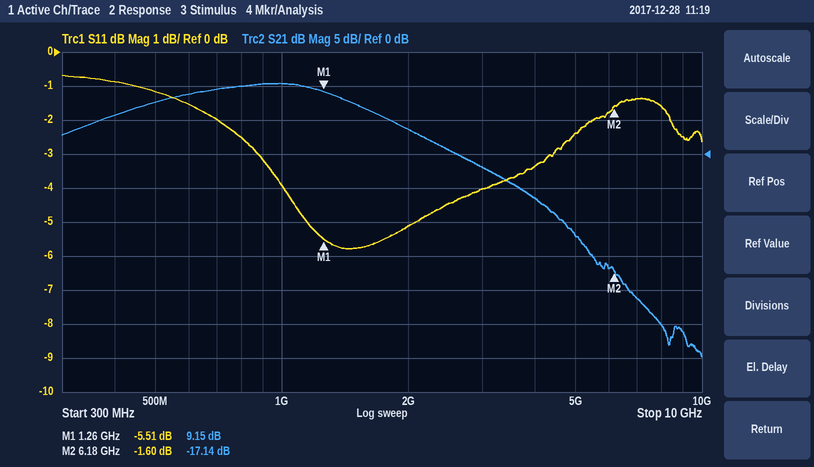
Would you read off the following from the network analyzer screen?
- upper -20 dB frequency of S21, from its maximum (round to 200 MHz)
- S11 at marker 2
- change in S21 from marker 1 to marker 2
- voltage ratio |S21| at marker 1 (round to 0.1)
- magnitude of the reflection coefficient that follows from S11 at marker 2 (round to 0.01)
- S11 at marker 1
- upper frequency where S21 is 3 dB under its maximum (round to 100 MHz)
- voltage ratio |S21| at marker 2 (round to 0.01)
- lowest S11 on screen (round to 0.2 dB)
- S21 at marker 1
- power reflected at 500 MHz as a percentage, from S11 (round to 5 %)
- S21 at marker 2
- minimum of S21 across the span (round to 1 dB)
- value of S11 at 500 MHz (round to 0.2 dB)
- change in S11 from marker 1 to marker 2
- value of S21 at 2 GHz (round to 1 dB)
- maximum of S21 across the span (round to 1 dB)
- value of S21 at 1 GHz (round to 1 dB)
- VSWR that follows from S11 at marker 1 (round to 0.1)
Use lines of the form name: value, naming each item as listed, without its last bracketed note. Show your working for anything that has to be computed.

upper -20 dB frequency of S21, from its maximum: 4.6 GHz
S11 at marker 2: -1.60 dB
change in S21 from marker 1 to marker 2: -17.14 − (9.15) = -26.29 dB
voltage ratio |S21| at marker 1: 10^(9.15/20) ≈ 2.9
magnitude of the reflection coefficient that follows from S11 at marker 2: 10^(-1.6/20) ≈ 0.83
S11 at marker 1: -5.51 dB
upper frequency where S21 is 3 dB under its maximum: 1.5 GHz
voltage ratio |S21| at marker 2: 10^(-17.14/20) ≈ 0.14
lowest S11 on screen: -5.8 dB
S21 at marker 1: 9.15 dB
power reflected at 500 MHz as a percentage, from S11: 10^(-1.2/10) ≈ 75.9 %, so 75 % to the nearest 5 %
S21 at marker 2: -17.14 dB
minimum of S21 across the span: -30 dB
value of S11 at 500 MHz: -1.2 dB
change in S11 from marker 1 to marker 2: -1.6 − (-5.51) = 3.91 dB
value of S21 at 2 GHz: 4 dB
maximum of S21 across the span: 10 dB
value of S21 at 1 GHz: 10 dB
VSWR that follows from S11 at marker 1: (1 + 0.5303)/(1 − 0.5303) ≈ 3.3
